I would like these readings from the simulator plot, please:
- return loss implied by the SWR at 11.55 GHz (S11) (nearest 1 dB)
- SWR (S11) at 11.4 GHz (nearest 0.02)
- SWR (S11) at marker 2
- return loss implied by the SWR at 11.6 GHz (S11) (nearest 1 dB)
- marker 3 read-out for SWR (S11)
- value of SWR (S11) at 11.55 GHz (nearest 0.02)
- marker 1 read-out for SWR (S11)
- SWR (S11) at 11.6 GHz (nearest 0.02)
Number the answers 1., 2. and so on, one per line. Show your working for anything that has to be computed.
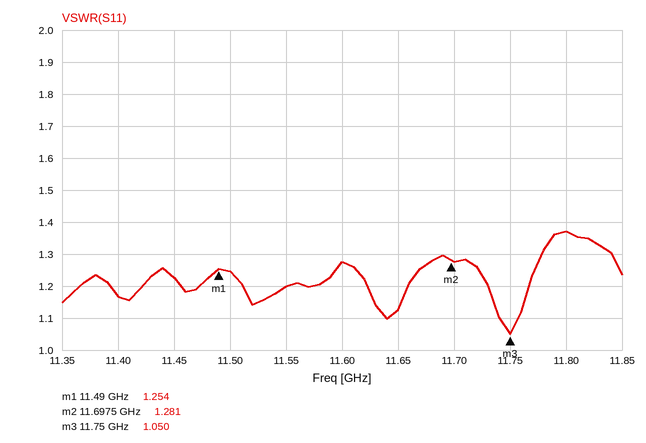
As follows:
1. −20 log10((1.2 − 1)/(1.2 + 1)) ≈ 21 dB
2. 1.16
3. 1.281
4. −20 log10((1.28 − 1)/(1.28 + 1)) ≈ 18 dB
5. 1.050
6. 1.20
7. 1.254
8. 1.28
